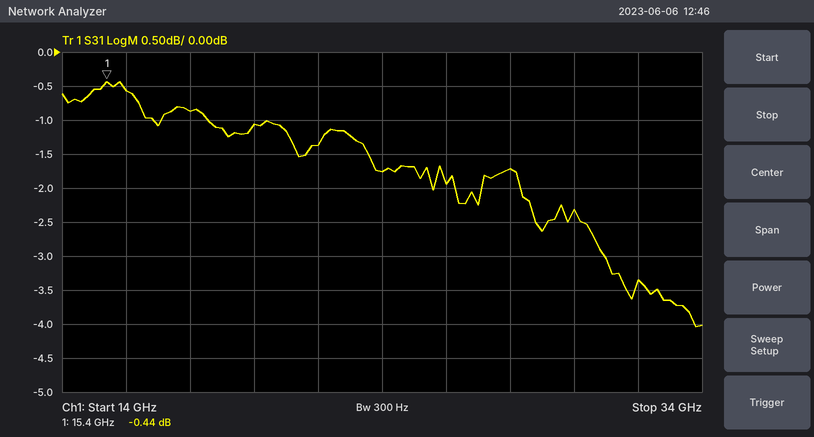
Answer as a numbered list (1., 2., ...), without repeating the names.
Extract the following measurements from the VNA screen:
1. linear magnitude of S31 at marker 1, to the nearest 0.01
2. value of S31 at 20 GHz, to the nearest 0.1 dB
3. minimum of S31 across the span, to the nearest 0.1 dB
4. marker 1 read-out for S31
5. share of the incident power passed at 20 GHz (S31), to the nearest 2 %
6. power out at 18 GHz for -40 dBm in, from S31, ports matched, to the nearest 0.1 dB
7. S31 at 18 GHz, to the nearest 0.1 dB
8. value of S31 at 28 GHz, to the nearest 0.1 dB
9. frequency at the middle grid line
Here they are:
1. 0.95
2. -1.1 dB
3. -4.0 dB
4. -0.44 dB
5. 78 %
6. -40.9 dBm
7. -0.9 dB
8. -1.7 dB
9. 24 GHz
